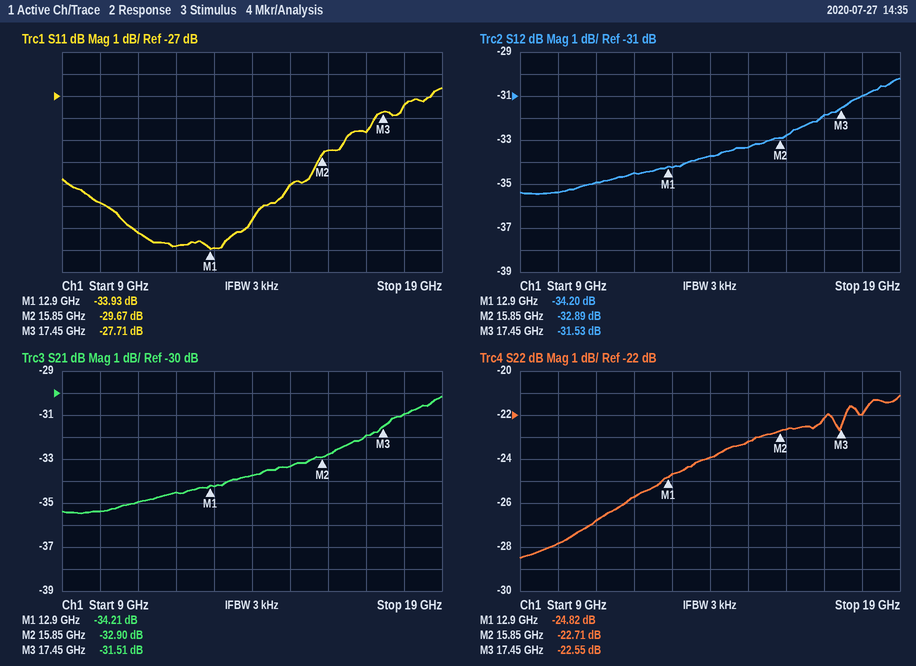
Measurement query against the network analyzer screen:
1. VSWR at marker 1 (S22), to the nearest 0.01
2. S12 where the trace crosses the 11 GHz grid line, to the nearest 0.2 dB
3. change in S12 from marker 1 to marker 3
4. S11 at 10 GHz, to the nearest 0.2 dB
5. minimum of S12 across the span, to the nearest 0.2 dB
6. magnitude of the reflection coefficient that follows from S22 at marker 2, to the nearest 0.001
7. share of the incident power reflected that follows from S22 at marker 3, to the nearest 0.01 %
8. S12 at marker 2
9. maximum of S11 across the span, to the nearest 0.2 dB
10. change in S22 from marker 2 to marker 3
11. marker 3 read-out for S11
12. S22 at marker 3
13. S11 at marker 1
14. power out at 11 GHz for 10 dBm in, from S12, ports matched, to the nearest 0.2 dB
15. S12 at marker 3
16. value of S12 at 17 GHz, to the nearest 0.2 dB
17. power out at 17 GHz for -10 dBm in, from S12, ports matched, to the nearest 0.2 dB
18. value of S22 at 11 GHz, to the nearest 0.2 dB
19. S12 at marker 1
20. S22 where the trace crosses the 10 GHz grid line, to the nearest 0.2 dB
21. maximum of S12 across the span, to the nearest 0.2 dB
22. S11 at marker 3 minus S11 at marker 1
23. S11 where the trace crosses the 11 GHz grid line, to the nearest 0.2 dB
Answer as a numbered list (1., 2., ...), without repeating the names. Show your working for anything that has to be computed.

1. (1 + 0.0574)/(1 − 0.0574) ≈ 1.12
2. -35.0 dB
3. -31.53 − (-34.2) = 2.67 dB
4. -31.8 dB
5. -35.4 dB
6. 10^(-22.71/20) ≈ 0.073
7. 10^(-22.55/10) ≈ 0.56 %
8. -32.89 dB
9. -26.6 dB
10. -22.55 − (-22.71) = 0.16 dB
11. -27.71 dB
12. -22.55 dB
13. -33.93 dB
14. 10 dBm + (-35.0 dB) = -25.0 dBm
15. -31.53 dB
16. -31.8 dB
17. -10 dBm + (-31.8 dB) = -41.8 dBm
18. -26.8 dB
19. -34.20 dB
20. -27.8 dB
21. -30.2 dB
22. -27.71 − (-33.93) = 6.22 dB
23. -33.2 dB
